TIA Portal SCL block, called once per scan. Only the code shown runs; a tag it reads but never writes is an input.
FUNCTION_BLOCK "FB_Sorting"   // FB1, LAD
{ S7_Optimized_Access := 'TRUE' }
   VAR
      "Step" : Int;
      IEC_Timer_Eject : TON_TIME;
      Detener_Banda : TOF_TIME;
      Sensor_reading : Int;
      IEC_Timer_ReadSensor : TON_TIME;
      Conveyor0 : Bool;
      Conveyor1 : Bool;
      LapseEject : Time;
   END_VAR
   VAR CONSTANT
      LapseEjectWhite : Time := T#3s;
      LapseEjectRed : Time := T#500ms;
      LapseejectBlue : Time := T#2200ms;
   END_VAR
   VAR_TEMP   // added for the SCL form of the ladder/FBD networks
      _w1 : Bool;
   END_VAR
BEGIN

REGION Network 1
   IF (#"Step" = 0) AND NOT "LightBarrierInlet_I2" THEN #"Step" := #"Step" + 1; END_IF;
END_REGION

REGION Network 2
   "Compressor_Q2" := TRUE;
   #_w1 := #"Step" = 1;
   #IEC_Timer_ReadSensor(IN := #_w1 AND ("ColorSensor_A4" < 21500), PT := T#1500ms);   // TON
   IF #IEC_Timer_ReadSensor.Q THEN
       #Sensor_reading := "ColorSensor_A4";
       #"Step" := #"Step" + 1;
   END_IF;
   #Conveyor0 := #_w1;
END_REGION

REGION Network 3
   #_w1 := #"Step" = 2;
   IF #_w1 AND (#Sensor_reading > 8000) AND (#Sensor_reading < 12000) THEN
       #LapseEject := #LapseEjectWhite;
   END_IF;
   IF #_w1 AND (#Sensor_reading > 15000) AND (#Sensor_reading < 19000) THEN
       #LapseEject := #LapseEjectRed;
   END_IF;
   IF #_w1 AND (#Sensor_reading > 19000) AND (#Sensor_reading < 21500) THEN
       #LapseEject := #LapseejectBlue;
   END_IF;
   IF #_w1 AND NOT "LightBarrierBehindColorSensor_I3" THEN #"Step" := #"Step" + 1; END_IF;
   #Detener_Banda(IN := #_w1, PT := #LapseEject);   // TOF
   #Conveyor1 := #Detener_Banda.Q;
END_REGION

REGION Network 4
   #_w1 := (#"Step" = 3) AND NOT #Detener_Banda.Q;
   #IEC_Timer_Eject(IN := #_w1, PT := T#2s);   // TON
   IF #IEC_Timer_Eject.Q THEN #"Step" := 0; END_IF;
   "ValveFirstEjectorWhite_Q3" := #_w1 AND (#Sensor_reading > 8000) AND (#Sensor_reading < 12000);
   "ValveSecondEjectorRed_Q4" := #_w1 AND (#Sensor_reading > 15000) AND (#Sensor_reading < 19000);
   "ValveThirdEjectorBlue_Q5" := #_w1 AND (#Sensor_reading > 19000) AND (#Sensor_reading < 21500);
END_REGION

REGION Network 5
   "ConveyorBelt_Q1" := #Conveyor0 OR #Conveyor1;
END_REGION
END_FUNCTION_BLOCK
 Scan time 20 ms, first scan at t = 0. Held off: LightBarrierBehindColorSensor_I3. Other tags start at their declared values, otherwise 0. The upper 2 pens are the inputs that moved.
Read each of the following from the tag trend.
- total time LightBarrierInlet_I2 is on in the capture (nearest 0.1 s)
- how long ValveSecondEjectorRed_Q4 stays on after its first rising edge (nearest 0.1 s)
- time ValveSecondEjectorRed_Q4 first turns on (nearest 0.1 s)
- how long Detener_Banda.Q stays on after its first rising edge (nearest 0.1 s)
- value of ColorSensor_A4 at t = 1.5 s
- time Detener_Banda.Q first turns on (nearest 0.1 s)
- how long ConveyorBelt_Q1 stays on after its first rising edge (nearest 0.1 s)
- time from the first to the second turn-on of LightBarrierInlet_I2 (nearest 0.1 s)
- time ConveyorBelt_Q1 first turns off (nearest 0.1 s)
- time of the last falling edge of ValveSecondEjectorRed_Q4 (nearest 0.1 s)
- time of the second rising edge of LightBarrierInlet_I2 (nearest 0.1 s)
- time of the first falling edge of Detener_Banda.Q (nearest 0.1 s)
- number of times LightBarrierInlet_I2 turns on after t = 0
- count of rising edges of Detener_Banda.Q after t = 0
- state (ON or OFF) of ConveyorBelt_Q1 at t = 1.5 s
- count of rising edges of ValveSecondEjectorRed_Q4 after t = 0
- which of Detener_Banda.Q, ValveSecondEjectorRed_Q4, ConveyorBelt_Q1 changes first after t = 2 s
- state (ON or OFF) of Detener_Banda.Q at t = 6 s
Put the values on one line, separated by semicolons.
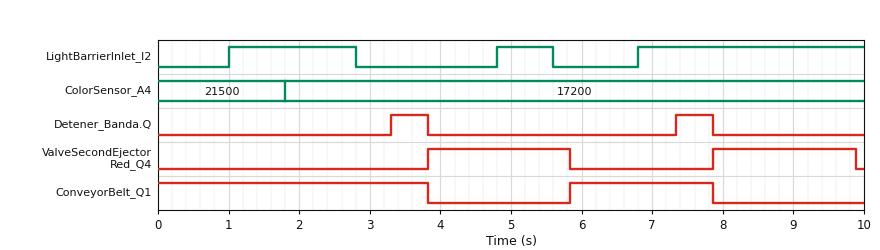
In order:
5.8 s; 2.0 s; 3.8 s; 0.5 s; 21500; 3.3 s; 2.0 s; 3.8 s; 3.8 s; 9.9 s; 4.8 s; 3.8 s; 3; 2; ON; 2; Detener_Banda.Q; OFF
